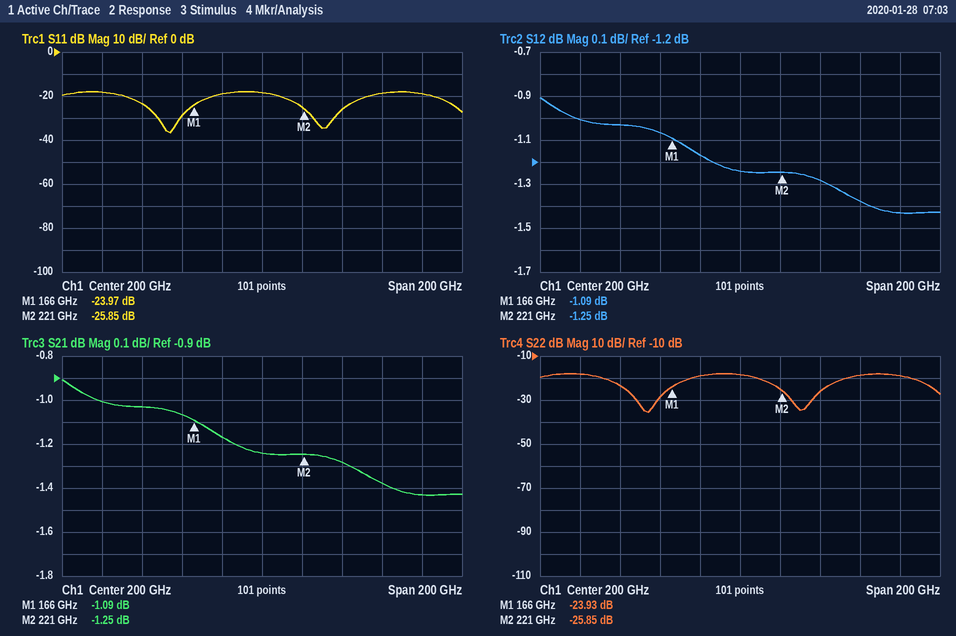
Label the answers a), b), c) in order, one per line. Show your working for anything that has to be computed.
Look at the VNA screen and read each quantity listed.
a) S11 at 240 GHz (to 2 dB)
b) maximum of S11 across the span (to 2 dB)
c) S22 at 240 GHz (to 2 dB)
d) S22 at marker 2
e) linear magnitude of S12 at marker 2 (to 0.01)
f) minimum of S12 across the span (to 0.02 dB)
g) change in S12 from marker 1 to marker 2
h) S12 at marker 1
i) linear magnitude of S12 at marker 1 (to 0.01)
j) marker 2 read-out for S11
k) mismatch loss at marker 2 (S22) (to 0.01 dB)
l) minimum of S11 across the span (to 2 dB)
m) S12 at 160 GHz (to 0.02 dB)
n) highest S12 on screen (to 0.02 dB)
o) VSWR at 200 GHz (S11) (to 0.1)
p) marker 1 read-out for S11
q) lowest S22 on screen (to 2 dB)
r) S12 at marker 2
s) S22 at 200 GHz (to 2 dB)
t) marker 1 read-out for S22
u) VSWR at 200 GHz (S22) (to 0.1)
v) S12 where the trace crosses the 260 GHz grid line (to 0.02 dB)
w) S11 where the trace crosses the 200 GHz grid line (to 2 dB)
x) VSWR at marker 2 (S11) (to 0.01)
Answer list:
a) -26 dB
b) -18 dB
c) -26 dB
d) -25.85 dB
e) 10^(-1.25/20) ≈ 0.87
f) -1.44 dB
g) -1.25 − (-1.09) = -0.16 dB
h) -1.09 dB
i) 10^(-1.09/20) ≈ 0.88
j) -25.85 dB
k) −10 log10(1 − 10^(-25.85/10)) ≈ 0.01 dB
l) -36 dB
m) -1.06 dB
n) -0.90 dB
o) |Γ| = 10^(-18/20) = 0.1259; VSWR = (1 + 0.1259)/(1 − 0.1259) ≈ 1.3
p) -23.97 dB
q) -36 dB
r) -1.25 dB
s) -18 dB
t) -23.93 dB
u) |Γ| = 10^(-18/20) = 0.1259; VSWR = (1 + 0.1259)/(1 − 0.1259) ≈ 1.3
v) -1.38 dB
w) -18 dB
x) (1 + 0.0510)/(1 − 0.0510) ≈ 1.11
